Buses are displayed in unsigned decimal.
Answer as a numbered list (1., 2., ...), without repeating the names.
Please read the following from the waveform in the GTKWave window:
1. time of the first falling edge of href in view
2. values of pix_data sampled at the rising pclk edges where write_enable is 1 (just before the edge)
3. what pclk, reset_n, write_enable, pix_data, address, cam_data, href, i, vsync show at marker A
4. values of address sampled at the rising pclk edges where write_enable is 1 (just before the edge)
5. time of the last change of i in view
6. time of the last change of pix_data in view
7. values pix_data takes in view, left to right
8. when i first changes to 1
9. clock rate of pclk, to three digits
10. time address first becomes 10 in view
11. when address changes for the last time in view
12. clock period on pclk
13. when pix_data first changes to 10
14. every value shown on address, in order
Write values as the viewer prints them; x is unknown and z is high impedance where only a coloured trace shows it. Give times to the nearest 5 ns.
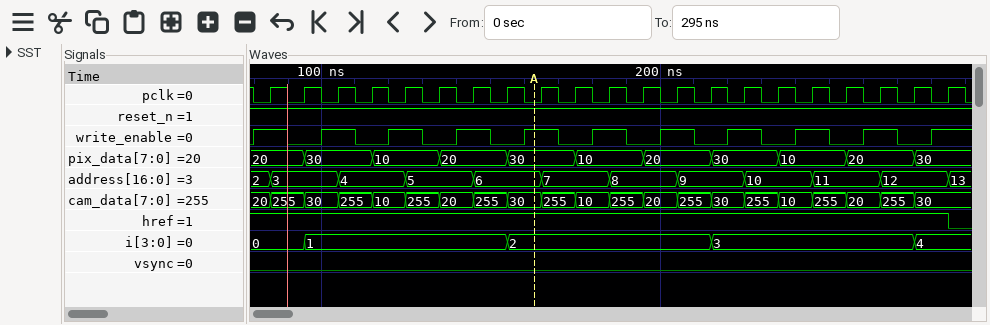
1. 285 ns
2. 20, 30, 10, 20, 30, 10, 20, 30, 10, 20, 30
3. pclk=0, reset_n=1, write_enable=1, pix_data=30, address=6, cam_data=30, href=1, i=2, vsync=0
4. 2, 3, 4, 5, 6, 7, 8, 9, 10, 11, 12
5. 275 ns
6. 275 ns
7. 20, 30, 10, 20, 30, 10, 20, 30, 10, 20, 30
8. 95 ns
9. 100 MHz
10. 225 ns
11. 285 ns
12. 10 ns
13. 115 ns
14. 2, 3, 4, 5, 6, 7, 8, 9, 10, 11, 12, 13
